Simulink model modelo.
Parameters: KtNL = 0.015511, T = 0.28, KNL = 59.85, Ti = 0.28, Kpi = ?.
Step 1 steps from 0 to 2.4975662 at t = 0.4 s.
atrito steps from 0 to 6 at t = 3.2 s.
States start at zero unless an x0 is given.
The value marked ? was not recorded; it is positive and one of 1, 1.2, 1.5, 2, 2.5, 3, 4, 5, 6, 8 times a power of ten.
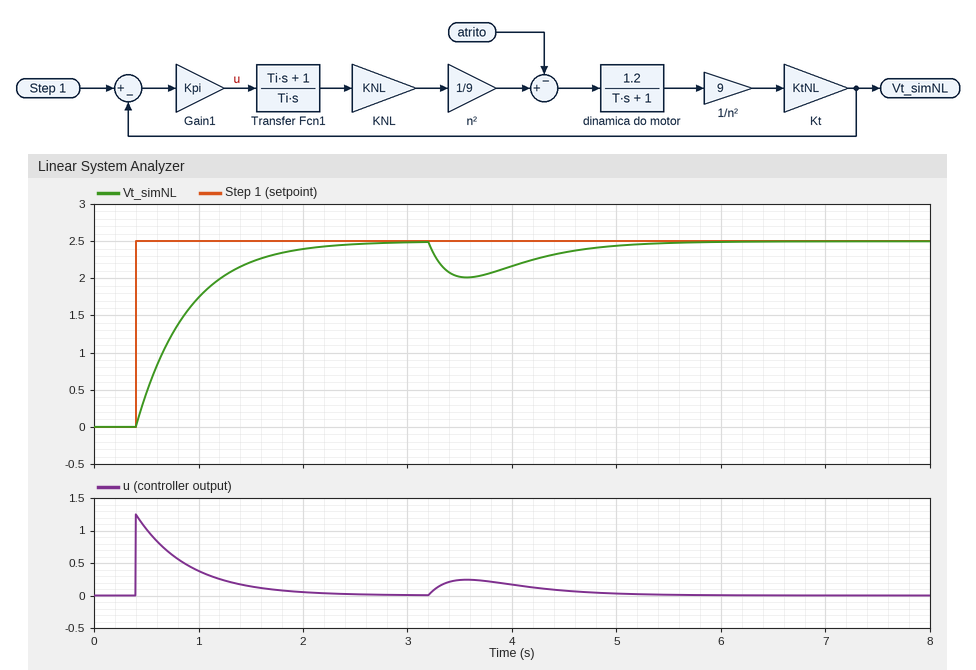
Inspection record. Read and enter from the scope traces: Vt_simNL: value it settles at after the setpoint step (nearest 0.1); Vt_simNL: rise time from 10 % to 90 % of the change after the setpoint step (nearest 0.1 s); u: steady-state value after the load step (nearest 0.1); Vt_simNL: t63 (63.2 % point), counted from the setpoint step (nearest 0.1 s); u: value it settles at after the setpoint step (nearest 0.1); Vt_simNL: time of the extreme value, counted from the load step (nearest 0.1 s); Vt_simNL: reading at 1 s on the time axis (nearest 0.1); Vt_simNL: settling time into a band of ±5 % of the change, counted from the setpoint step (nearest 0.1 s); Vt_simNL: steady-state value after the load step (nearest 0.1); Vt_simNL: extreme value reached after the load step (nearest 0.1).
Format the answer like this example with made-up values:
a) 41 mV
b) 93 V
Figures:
a) 2.5
b) 1.1 s
c) 0.0
d) 0.5 s
e) 0.0
f) 0.4 s
g) 1.7
h) 1.5 s
i) 2.5
j) 2.0
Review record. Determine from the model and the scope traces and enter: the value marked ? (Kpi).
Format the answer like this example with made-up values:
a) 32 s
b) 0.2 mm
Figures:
a) 0.5
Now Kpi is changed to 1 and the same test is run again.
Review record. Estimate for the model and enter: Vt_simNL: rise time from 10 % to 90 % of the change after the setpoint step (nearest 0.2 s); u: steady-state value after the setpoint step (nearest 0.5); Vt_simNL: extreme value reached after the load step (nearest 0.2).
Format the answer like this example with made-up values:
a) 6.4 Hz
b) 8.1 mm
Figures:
a) 0.6 s
b) 0.0
c) 2.2
